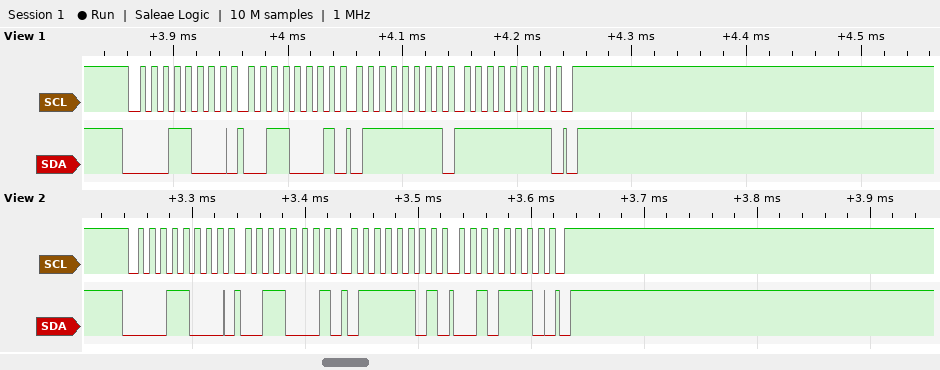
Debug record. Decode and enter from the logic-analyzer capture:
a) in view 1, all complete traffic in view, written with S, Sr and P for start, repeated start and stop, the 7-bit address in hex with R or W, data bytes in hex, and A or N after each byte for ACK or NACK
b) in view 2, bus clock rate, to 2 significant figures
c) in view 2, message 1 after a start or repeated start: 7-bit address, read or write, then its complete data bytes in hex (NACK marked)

S 0CW A 31 A 7F A FF A P
100 kHz
0x0C write: 31 7D 2E
